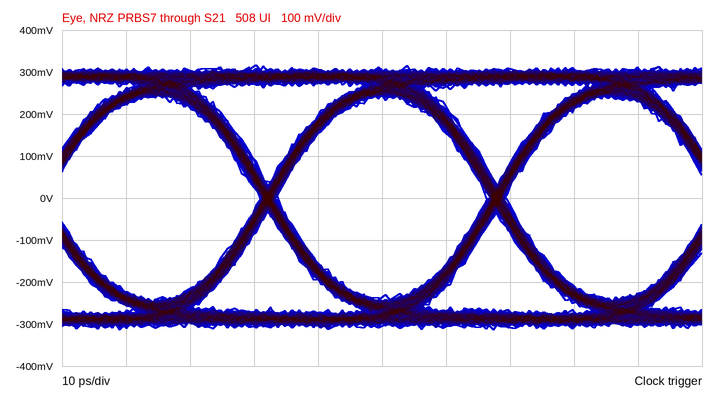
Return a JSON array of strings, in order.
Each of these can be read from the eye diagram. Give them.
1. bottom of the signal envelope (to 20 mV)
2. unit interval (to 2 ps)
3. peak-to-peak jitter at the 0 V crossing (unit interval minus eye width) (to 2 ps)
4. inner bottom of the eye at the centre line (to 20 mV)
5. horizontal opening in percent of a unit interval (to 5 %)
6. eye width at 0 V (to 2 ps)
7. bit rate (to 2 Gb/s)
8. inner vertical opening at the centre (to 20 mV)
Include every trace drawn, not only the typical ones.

["-320 mV", "36 ps", "4 ps", "-240 mV", "90 %", "32 ps", "28 Gb/s", "480 mV"]
